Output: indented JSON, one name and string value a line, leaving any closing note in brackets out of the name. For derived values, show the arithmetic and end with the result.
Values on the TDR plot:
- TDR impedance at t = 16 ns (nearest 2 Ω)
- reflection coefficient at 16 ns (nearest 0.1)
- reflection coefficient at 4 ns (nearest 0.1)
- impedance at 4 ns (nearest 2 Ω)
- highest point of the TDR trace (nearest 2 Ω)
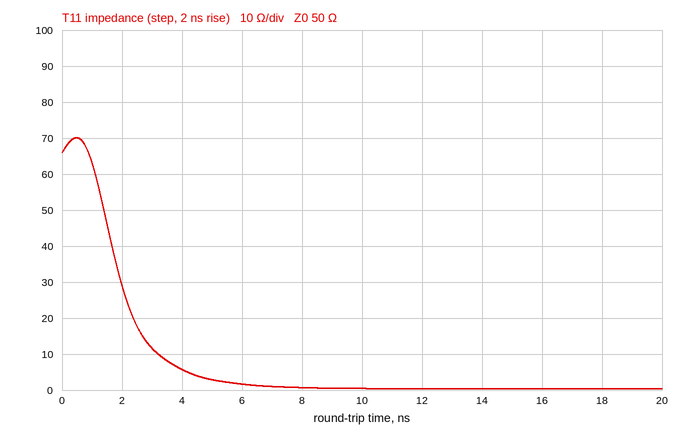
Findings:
{
  "TDR impedance at t = 16 ns": "0 Ω",
  "reflection coefficient at 16 ns": "(0 − 50)/(0 + 50) ≈ -1.0",
  "reflection coefficient at 4 ns": "(6 − 50)/(6 + 50) ≈ -0.8",
  "impedance at 4 ns": "6 Ω",
  "highest point of the TDR trace": "70 Ω"
}
